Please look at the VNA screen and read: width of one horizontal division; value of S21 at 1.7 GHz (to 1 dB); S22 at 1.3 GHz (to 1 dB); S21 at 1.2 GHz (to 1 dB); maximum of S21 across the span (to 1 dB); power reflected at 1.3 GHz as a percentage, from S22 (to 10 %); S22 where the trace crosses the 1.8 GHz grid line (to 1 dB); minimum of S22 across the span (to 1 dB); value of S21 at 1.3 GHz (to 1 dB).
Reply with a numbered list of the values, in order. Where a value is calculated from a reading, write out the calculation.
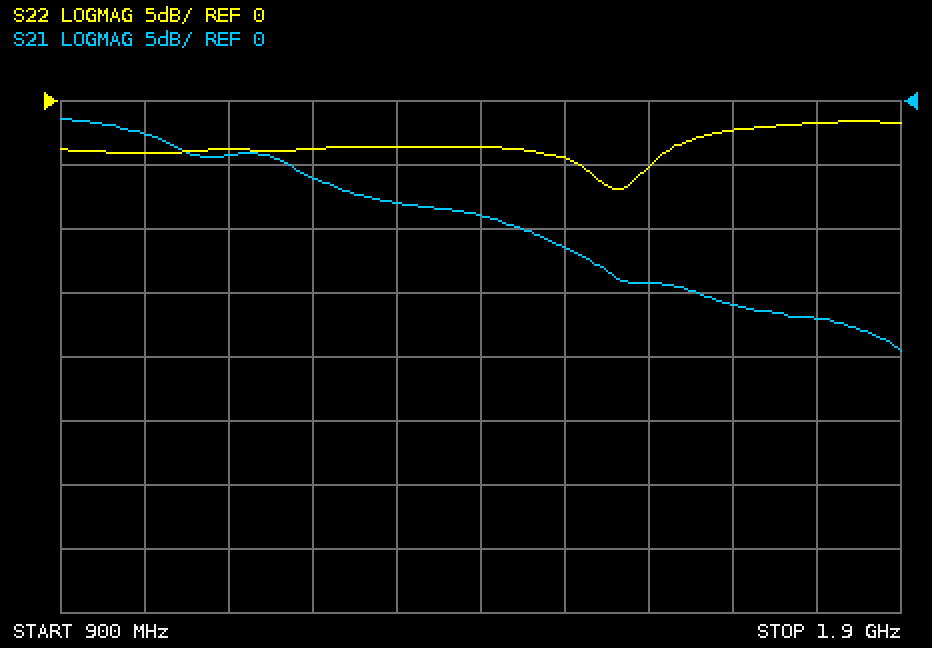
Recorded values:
1. 100 MHz
2. -16 dB
3. -4 dB
4. -6 dB
5. -1 dB
6. 10^(-4/10) ≈ 40 %
7. -2 dB
8. -7 dB
9. -8 dB
